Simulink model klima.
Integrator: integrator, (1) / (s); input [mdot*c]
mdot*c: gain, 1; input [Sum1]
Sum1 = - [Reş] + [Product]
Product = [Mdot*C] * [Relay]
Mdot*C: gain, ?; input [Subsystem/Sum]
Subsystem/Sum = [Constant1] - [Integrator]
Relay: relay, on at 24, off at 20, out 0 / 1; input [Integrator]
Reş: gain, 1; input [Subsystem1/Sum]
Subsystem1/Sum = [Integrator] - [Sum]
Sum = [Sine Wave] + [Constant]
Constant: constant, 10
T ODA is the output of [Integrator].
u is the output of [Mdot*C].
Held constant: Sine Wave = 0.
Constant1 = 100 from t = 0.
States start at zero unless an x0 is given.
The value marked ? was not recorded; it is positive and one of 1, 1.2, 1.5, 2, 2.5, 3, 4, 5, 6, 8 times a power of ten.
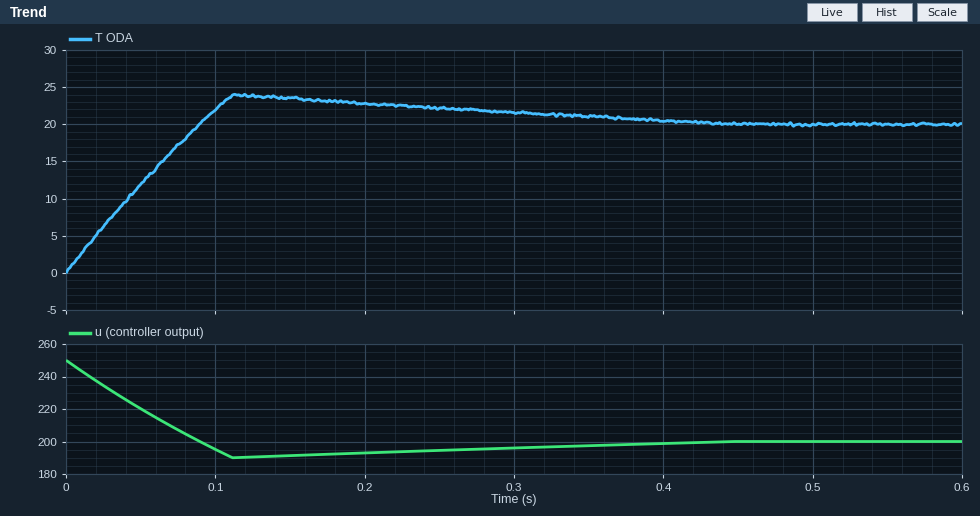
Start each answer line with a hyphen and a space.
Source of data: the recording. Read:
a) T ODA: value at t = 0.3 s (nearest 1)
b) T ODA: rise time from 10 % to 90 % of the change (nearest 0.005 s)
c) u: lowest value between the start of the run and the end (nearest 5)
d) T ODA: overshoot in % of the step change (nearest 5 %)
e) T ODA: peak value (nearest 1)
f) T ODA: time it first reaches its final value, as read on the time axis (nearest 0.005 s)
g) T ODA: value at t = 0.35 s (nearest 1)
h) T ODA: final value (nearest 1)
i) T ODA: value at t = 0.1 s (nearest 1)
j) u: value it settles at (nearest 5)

- 22
- 0.070 s
- 190
- 20 %
- 24
- 0.090 s
- 21
- 20
- 22
- 200
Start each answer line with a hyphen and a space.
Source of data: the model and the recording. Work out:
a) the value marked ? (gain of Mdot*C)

- 2.5
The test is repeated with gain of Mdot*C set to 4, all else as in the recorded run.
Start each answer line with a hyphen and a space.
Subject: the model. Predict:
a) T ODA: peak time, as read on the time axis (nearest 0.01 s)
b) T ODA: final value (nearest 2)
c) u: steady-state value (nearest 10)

- 0.07 s
- 20
- 320
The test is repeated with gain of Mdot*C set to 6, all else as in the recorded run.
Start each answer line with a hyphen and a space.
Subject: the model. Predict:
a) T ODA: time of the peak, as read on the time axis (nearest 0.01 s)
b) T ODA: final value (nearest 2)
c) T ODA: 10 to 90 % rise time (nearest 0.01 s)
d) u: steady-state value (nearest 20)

- 0.05 s
- 20
- 0.03 s
- 480
